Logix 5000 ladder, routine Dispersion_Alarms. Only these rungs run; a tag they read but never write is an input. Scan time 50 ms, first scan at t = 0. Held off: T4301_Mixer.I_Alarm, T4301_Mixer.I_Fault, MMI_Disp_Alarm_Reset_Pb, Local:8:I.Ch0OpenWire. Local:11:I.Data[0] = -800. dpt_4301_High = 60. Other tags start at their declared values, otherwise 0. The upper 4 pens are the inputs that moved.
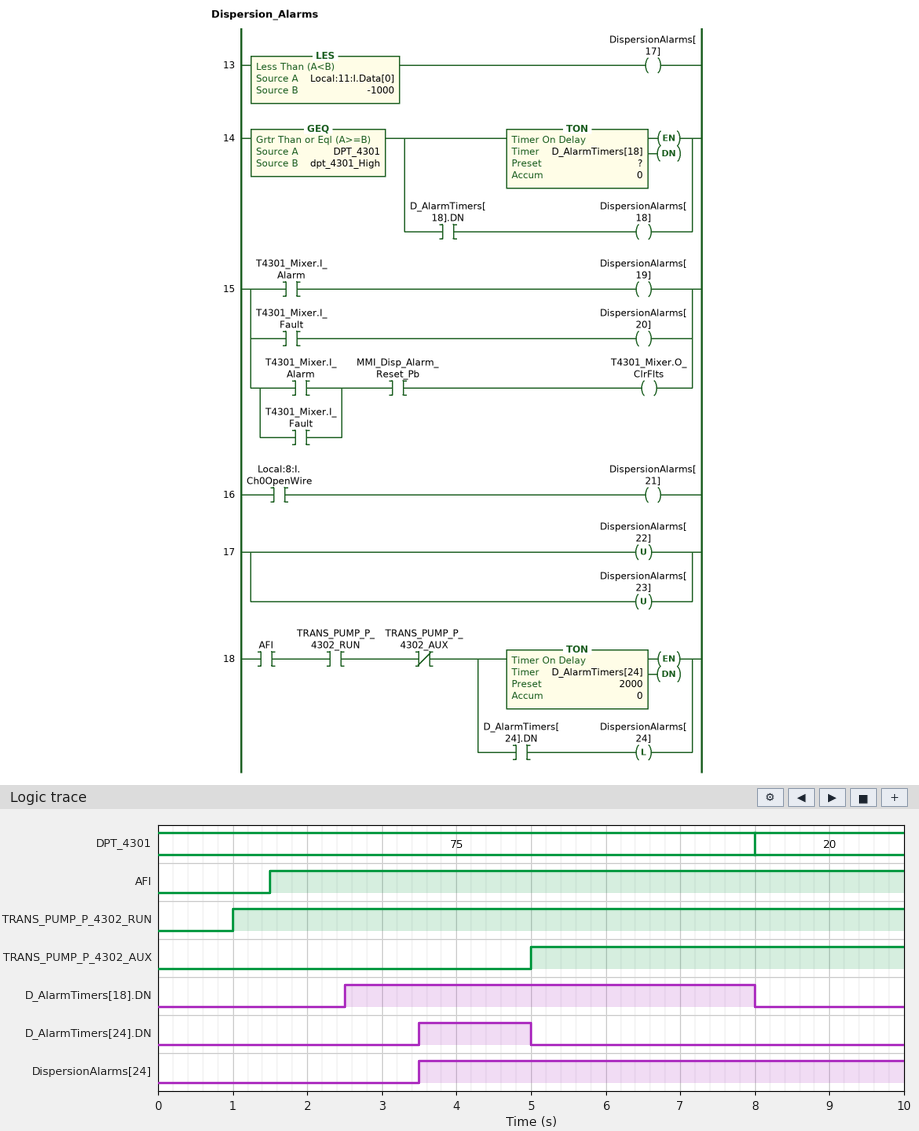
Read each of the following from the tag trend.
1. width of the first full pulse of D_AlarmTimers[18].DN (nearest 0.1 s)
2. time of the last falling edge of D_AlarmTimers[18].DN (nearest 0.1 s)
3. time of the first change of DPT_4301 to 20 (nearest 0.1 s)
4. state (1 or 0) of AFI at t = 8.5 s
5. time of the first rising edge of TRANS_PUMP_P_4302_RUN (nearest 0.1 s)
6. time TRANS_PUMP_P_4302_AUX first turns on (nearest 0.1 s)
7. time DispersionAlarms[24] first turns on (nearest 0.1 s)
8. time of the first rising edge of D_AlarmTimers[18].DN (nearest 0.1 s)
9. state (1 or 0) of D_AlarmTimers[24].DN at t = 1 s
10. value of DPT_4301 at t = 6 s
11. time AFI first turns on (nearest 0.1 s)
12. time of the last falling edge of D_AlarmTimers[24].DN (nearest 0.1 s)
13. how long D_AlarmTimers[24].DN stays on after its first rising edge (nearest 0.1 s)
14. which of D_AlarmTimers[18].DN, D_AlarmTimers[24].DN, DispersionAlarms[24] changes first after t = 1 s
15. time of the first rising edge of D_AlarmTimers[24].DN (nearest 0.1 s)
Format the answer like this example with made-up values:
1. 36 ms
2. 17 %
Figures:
1. 5.5 s
2. 8.0 s
3. 8.0 s
4. 1
5. 1.0 s
6. 5.0 s
7. 3.5 s
8. 2.5 s
9. 0
10. 75
11. 1.5 s
12. 5.0 s
13. 1.5 s
14. D_AlarmTimers[18].DN
15. 3.5 s
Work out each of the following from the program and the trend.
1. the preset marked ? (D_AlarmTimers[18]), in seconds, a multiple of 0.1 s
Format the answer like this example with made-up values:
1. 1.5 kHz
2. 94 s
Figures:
1. 2.5 s
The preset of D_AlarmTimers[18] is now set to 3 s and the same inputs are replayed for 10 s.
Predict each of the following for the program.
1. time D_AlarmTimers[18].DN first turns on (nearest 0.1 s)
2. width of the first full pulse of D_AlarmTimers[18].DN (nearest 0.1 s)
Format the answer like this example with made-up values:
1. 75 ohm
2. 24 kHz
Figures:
1. 3.0 s
2. 5.0 s
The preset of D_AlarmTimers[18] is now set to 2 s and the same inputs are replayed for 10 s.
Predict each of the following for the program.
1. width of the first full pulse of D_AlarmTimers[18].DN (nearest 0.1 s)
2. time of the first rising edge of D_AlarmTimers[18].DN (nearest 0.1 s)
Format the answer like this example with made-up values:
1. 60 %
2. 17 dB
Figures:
1. 6.0 s
2. 2.0 s
